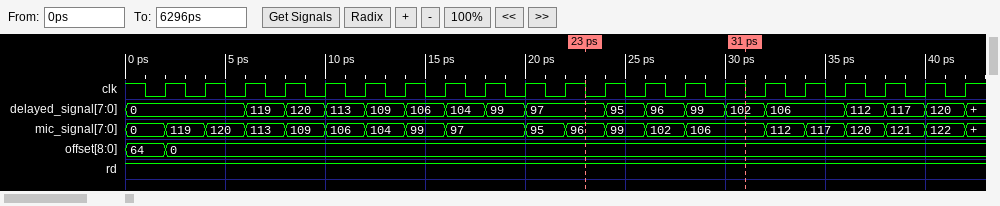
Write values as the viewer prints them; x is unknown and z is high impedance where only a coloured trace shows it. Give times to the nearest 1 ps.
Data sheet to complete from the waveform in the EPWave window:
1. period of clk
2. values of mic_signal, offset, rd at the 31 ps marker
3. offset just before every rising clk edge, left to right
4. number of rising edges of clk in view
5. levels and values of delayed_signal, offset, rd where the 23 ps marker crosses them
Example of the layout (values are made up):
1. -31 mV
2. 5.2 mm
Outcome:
1. 2 ps
2. mic_signal=106, offset=0, rd=1
3. 64, 0, 0, 0, 0, 0, 0, 0, 0, 0, 0, 0, 0, 0, 0, 0, 0, 0, 0, 0, 0
4. 21
5. delayed_signal=97, offset=0, rd=1
